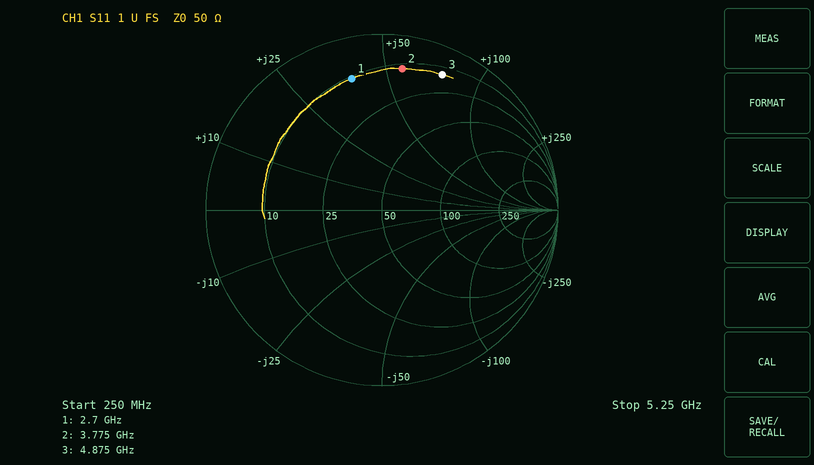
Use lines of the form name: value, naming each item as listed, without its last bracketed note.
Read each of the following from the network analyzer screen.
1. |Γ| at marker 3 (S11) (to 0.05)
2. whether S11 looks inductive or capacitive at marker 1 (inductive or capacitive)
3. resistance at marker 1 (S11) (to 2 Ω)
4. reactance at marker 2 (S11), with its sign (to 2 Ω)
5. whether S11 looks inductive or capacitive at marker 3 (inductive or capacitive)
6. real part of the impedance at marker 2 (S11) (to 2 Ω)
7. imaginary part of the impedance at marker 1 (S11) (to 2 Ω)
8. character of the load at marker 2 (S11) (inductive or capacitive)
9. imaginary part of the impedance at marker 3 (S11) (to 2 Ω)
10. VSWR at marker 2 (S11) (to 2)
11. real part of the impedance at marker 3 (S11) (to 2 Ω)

|Γ| at marker 3 (S11): 0.85
whether S11 looks inductive or capacitive at marker 1: inductive
resistance at marker 1 (S11): 10 Ω
reactance at marker 2 (S11), with its sign: +56 Ω
whether S11 looks inductive or capacitive at marker 3: inductive
real part of the impedance at marker 2 (S11): 12 Ω
imaginary part of the impedance at marker 1 (S11): +38 Ω
character of the load at marker 2 (S11): inductive
imaginary part of the impedance at marker 3 (S11): +76 Ω
VSWR at marker 2 (S11): 10
real part of the impedance at marker 3 (S11): 14 Ω
